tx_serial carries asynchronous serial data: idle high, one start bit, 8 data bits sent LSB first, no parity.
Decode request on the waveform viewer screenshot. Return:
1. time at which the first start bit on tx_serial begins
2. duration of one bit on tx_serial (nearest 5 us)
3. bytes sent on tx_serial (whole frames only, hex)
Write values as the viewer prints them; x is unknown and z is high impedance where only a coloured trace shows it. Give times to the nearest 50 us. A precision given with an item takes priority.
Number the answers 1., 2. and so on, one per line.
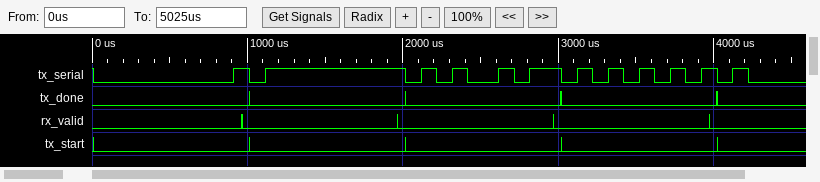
1. 0 us
2. 100 us
3. 00, FF, A5, 55
